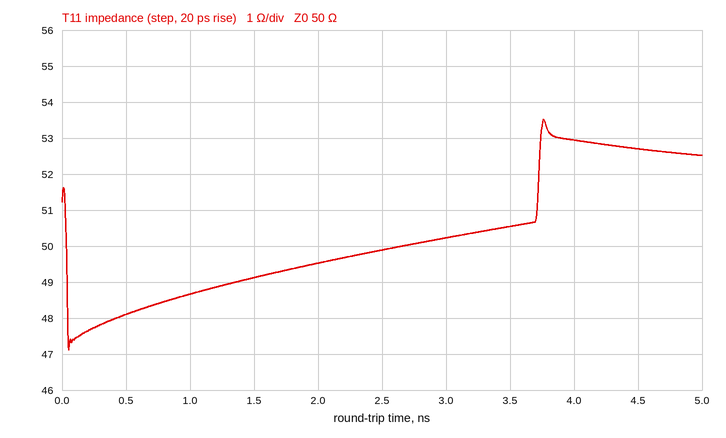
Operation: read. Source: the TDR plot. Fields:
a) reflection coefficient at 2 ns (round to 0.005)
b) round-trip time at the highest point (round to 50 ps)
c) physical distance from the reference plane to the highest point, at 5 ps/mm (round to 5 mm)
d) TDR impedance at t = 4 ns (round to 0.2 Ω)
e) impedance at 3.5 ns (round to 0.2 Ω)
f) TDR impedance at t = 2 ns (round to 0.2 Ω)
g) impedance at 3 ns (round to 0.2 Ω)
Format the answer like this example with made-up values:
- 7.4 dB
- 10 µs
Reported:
- -0.005
- 3.75 ns
- 375 mm
- 53.0 Ω
- 50.6 Ω
- 49.6 Ω
- 50.2 Ω
